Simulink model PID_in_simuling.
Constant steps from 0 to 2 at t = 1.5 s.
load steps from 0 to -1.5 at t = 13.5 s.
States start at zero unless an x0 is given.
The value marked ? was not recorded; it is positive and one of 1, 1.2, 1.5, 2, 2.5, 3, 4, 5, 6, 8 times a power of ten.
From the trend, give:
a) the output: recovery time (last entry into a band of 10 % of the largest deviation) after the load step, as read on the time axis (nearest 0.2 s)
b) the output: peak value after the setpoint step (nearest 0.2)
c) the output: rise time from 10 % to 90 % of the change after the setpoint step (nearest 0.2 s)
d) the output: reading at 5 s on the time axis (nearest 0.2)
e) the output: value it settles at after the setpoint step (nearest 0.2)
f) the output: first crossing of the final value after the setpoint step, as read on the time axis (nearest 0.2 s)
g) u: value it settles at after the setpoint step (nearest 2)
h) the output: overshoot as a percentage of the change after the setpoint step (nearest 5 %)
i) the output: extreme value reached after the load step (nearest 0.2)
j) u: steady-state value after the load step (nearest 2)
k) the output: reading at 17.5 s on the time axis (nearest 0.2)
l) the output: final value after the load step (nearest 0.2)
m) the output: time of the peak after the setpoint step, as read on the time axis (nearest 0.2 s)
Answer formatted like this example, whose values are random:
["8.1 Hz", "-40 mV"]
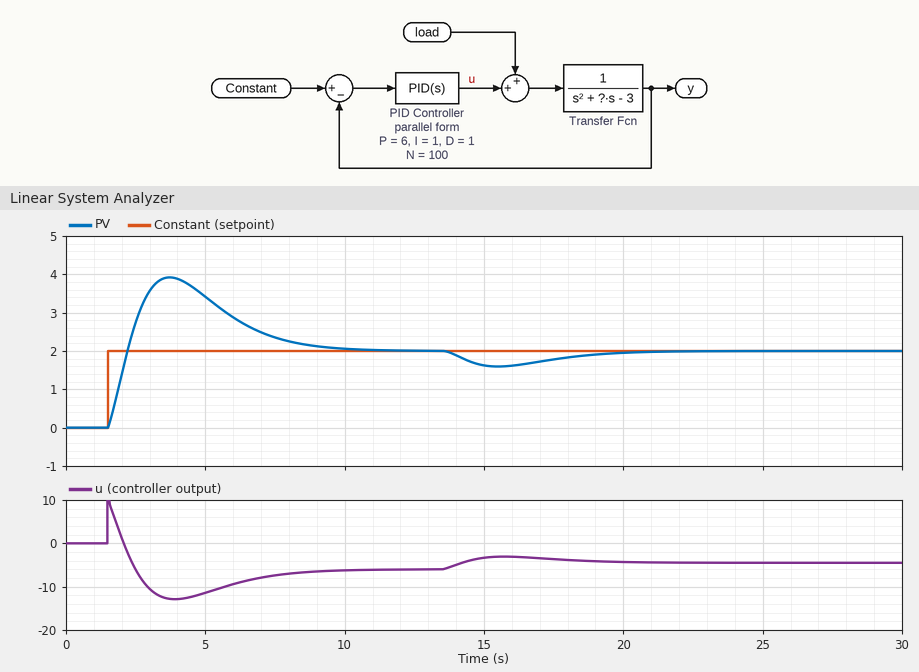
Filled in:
["20.2 s", "4.0", "0.6 s", "3.4", "2.0", "2.2 s", "-6", "95 %", "1.6", "-4", "1.8", "2.0", "3.8 s"]
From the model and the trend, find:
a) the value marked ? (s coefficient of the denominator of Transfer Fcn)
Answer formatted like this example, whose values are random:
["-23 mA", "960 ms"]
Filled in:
["2"]
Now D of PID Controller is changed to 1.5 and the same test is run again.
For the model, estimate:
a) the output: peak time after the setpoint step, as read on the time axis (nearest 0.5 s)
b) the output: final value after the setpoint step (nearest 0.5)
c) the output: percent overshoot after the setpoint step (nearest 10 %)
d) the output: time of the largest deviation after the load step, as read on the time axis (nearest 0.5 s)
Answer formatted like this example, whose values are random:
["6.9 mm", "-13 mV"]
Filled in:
["4.0 s", "2.0", "90 %", "15.5 s"]
